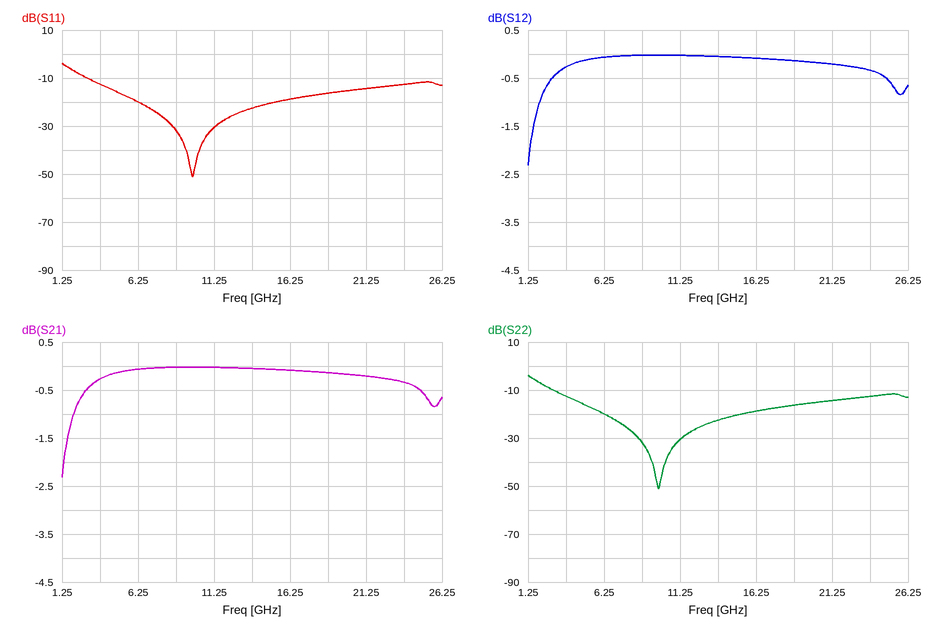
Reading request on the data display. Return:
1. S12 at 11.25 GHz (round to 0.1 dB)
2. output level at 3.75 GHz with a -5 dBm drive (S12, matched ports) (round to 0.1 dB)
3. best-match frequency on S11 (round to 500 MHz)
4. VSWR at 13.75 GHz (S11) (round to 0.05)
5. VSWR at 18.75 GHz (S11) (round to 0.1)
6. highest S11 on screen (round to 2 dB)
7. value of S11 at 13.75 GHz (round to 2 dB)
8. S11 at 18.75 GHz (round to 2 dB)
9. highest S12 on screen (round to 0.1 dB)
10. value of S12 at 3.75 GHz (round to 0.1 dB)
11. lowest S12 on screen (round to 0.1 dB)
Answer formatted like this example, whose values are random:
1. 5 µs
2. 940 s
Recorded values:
1. 0.0 dB
2. -5.3 dBm
3. 10.0 GHz
4. 1.15
5. 1.4
6. -4 dB
7. -22 dB
8. -16 dB
9. 0.0 dB
10. -0.3 dB
11. -2.3 dB
